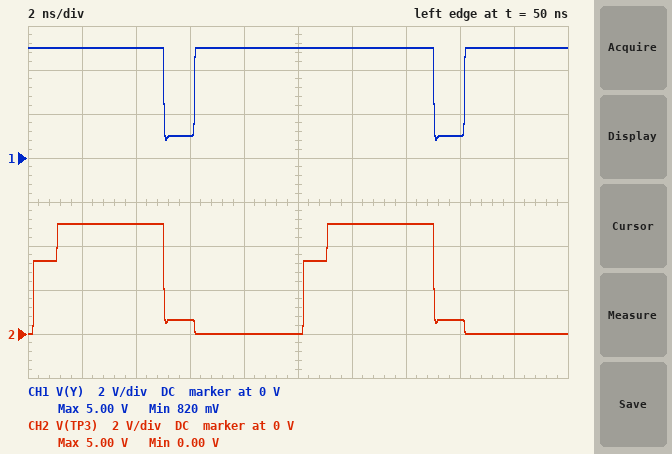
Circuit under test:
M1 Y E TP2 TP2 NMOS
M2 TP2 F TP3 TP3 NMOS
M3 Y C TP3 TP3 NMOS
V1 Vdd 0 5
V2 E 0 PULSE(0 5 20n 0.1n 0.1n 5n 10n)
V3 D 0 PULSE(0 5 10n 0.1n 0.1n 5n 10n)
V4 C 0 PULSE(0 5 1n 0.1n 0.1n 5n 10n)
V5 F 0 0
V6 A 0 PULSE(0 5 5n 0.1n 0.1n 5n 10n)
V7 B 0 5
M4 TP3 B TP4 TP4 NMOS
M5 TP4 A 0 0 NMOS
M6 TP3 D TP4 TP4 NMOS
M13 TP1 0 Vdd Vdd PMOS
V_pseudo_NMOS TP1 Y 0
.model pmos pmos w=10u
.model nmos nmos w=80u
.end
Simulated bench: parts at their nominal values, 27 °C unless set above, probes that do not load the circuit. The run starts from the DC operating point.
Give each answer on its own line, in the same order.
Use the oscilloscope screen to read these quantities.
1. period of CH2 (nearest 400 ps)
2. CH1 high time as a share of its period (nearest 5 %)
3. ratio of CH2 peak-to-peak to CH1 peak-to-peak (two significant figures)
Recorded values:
10.0 ns
90 %
1.2
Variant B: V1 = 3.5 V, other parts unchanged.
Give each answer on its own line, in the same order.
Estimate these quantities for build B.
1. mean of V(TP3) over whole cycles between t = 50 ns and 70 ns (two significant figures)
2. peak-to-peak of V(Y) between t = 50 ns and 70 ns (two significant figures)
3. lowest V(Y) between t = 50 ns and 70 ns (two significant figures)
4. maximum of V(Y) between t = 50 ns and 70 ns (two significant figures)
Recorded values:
1.6 V
3.1 V
390 mV
3.5 V
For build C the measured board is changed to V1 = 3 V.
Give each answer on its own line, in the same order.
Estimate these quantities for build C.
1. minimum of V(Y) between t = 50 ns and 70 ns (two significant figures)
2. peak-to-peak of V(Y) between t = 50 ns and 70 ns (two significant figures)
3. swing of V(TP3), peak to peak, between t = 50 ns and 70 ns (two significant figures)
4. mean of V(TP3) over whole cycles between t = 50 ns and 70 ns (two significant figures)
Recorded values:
290 mV
2.7 V
3.0 V
1.4 V
